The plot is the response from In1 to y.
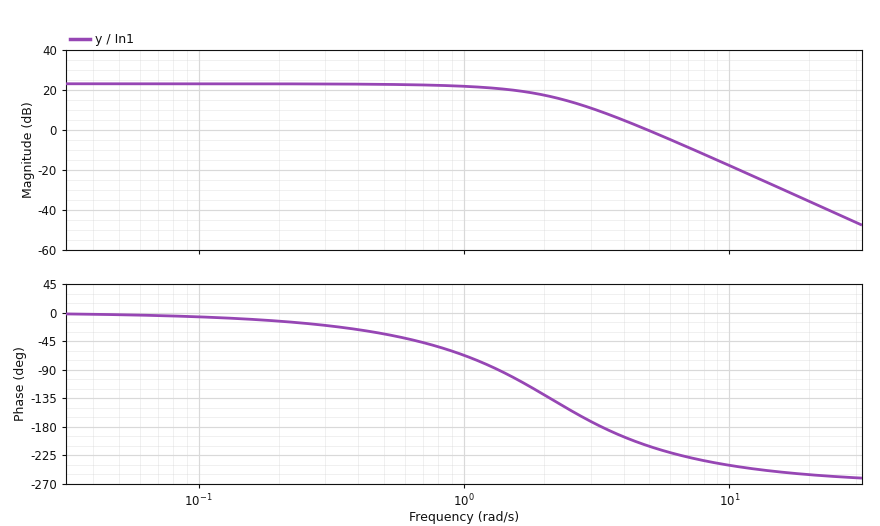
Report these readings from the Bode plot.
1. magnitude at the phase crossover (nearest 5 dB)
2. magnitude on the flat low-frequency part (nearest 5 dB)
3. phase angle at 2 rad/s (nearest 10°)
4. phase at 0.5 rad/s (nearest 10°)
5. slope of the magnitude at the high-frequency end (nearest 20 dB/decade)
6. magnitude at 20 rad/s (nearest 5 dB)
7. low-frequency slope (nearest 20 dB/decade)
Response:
10 dB
25 dB
-130°
-30°
-60 dB/decade
-35 dB
0 dB/decade
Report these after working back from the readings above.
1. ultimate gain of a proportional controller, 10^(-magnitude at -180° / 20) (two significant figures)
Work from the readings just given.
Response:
0.32
